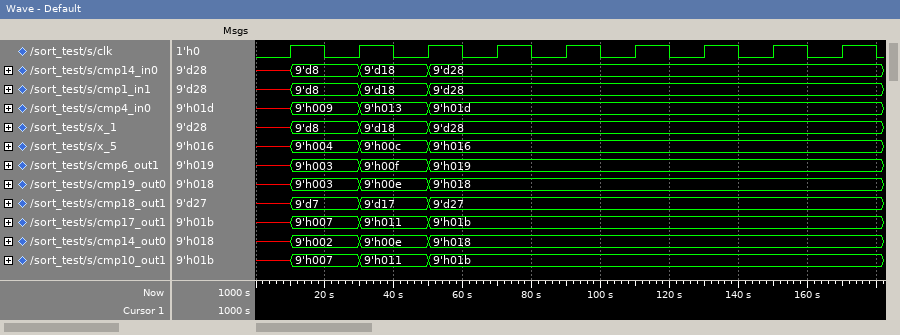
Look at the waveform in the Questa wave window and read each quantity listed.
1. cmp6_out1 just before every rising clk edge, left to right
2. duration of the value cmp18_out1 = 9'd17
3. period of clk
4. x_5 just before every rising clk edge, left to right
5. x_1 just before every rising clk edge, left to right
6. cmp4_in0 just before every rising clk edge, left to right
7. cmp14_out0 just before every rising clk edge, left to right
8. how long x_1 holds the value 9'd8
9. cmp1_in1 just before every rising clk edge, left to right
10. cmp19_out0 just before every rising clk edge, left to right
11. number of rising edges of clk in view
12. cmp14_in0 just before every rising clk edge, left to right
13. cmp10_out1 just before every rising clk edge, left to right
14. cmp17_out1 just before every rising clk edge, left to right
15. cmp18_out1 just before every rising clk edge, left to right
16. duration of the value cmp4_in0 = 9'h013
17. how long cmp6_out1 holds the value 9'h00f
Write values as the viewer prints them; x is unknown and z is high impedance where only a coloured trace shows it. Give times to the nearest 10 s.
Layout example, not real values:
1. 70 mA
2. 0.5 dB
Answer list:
1. x, 9'h003, 9'h00f, 9'h019, 9'h019, 9'h019, 9'h019, 9'h019, 9'h019
2. 20 s
3. 20 s
4. x, 9'h004, 9'h00c, 9'h016, 9'h016, 9'h016, 9'h016, 9'h016, 9'h016
5. x, 9'd8, 9'd18, 9'd28, 9'd28, 9'd28, 9'd28, 9'd28, 9'd28
6. x, 9'h009, 9'h013, 9'h01d, 9'h01d, 9'h01d, 9'h01d, 9'h01d, 9'h01d
7. x, 9'h002, 9'h00e, 9'h018, 9'h018, 9'h018, 9'h018, 9'h018, 9'h018
8. 20 s
9. x, 9'd8, 9'd18, 9'd28, 9'd28, 9'd28, 9'd28, 9'd28, 9'd28
10. x, 9'h003, 9'h00e, 9'h018, 9'h018, 9'h018, 9'h018, 9'h018, 9'h018
11. 9
12. x, 9'd8, 9'd18, 9'd28, 9'd28, 9'd28, 9'd28, 9'd28, 9'd28
13. x, 9'h007, 9'h011, 9'h01b, 9'h01b, 9'h01b, 9'h01b, 9'h01b, 9'h01b
14. x, 9'h007, 9'h011, 9'h01b, 9'h01b, 9'h01b, 9'h01b, 9'h01b, 9'h01b
15. x, 9'd7, 9'd17, 9'd27, 9'd27, 9'd27, 9'd27, 9'd27, 9'd27
16. 20 s
17. 20 s
